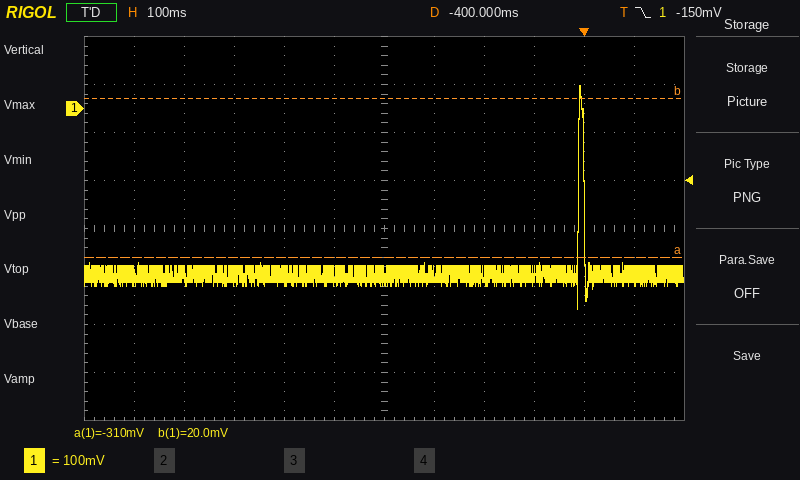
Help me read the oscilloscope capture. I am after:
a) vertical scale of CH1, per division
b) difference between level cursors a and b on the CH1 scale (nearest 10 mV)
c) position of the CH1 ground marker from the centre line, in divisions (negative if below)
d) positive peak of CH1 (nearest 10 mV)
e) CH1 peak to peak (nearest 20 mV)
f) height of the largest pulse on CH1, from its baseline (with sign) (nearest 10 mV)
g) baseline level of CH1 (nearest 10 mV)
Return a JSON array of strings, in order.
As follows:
["100 mV", "330 mV", "+2.5 div", "50 mV", "460 mV", "+390 mV", "-340 mV"]
